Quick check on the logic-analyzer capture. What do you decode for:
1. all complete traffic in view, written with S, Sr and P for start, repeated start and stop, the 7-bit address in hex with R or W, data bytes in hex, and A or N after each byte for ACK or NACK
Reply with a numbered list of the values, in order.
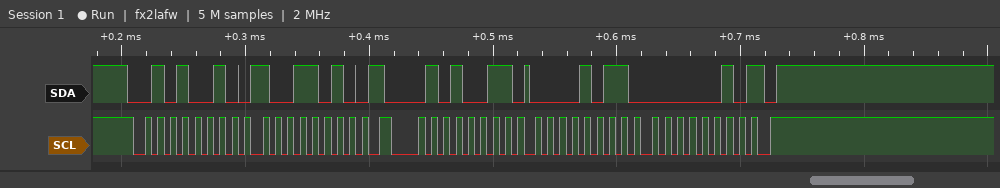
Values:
1. S 29W A 9A A Sr 29R A 0B A 02 N P
